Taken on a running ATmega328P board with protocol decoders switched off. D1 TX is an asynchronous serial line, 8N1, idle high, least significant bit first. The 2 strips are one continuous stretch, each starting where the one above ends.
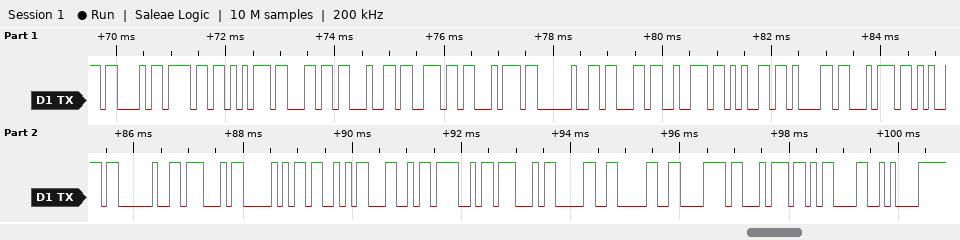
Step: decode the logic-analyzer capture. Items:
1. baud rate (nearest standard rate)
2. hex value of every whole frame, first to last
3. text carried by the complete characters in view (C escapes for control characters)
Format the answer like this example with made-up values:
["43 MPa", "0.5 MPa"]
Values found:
["9600 baud", "43 6F 75 6C 64 6E 74 20 63 72 65 61 74 65 20 47 50 53 4C 4F 47 30 30 78 74 0D 0A", "\"Couldnt create GPSLOG00xt\\r\\n\""]
